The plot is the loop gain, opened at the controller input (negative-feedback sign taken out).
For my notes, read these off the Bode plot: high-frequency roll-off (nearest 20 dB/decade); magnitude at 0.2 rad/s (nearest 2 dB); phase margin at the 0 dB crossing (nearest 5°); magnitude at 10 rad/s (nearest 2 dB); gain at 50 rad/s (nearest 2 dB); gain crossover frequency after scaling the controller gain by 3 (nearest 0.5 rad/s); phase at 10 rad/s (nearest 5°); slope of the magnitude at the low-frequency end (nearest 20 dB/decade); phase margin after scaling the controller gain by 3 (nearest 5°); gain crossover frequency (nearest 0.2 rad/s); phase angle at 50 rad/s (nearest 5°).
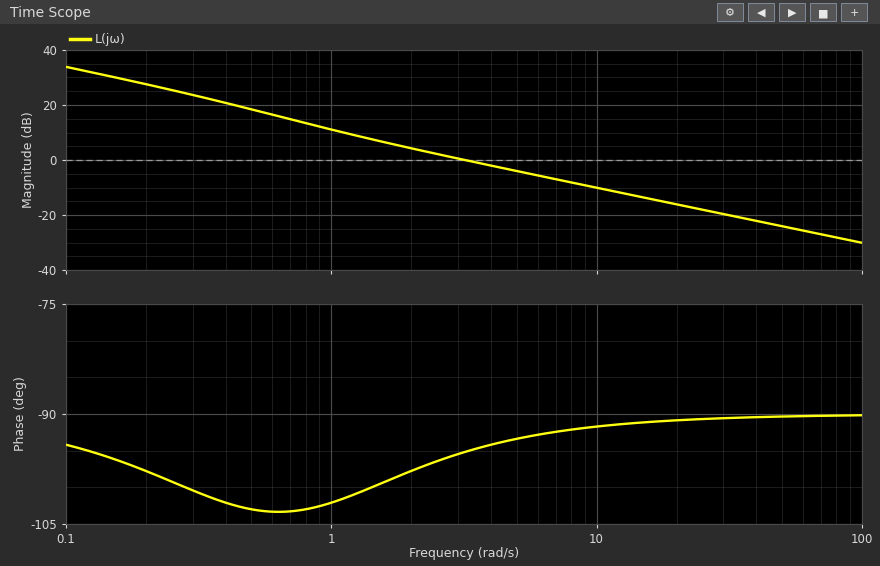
-20 dB/decade
28 dB
85°
-10 dB
-24 dB
9.5 rad/s
-90°
-20 dB/decade
90°
3.2 rad/s
-90°
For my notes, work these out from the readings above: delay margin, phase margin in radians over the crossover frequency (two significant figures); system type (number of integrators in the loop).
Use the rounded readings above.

0.46 s
1
